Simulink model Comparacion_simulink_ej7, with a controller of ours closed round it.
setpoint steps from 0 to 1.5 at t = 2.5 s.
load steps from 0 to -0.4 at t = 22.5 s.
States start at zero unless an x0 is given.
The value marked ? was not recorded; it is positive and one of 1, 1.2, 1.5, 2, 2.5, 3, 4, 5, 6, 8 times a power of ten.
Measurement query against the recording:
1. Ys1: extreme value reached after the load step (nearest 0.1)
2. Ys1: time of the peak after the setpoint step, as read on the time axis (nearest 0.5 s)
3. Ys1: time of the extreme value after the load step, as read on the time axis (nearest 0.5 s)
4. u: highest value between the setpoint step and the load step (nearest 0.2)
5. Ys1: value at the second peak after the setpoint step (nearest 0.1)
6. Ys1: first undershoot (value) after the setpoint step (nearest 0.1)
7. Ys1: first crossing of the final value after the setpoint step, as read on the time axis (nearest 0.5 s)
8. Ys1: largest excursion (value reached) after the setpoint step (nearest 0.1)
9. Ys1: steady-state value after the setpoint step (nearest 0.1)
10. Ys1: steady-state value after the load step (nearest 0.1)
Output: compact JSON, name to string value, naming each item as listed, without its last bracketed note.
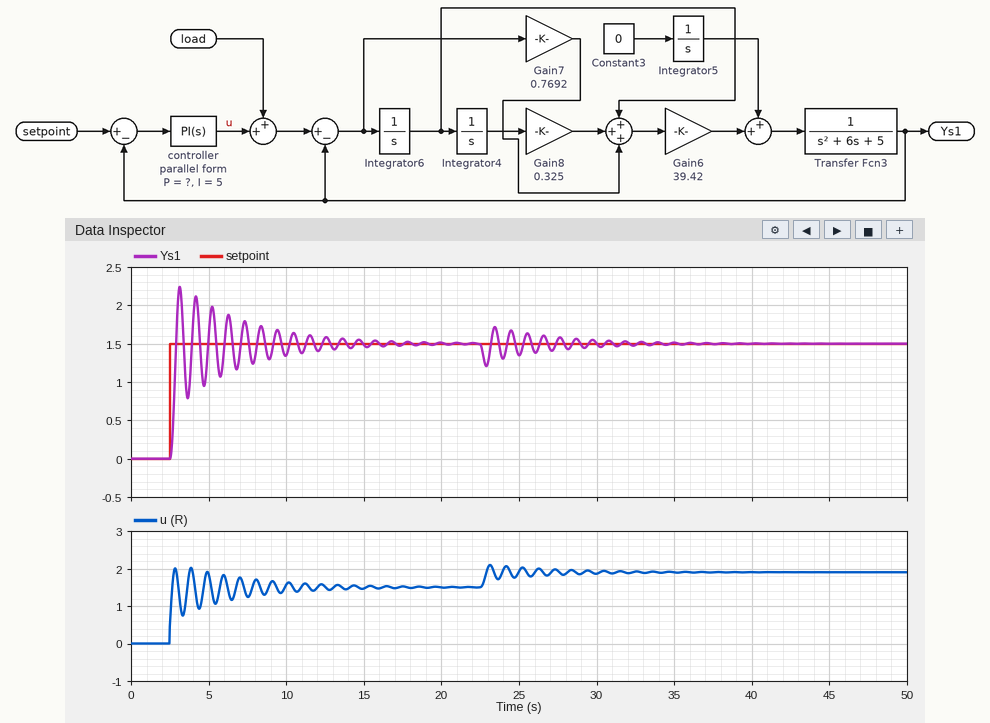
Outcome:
{"Ys1: extreme value reached after the load step": "1.2", "Ys1: time of the peak after the setpoint step, as read on the time axis": "3.0 s", "Ys1: time of the extreme value after the load step, as read on the time axis": "23.0 s", "u: highest value between the setpoint step and the load step": "2.0", "Ys1: value at the second peak after the setpoint step": "2.1", "Ys1: first undershoot (value) after the setpoint step": "0.8", "Ys1: first crossing of the final value after the setpoint step, as read on the time axis": "3.0 s", "Ys1: largest excursion (value reached) after the setpoint step": "2.2", "Ys1: steady-state value after the setpoint step": "1.5", "Ys1: steady-state value after the load step": "1.5"}
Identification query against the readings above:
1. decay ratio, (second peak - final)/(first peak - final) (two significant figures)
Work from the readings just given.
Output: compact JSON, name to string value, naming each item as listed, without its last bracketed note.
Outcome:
{"decay ratio, (second peak - final)/(first peak - final)": "0.86"}
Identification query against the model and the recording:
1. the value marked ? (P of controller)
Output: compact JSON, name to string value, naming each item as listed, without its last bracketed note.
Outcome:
{"the value marked ?": "0.3"}
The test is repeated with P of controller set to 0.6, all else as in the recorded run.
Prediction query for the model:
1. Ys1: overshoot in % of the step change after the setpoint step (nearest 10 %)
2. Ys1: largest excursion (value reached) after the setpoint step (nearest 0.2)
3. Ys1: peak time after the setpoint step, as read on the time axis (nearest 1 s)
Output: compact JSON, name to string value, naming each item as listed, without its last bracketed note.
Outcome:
{"Ys1: overshoot in % of the step change after the setpoint step": "40 %", "Ys1: largest excursion (value reached) after the setpoint step": "2.0", "Ys1: peak time after the setpoint step, as read on the time axis": "3 s"}
